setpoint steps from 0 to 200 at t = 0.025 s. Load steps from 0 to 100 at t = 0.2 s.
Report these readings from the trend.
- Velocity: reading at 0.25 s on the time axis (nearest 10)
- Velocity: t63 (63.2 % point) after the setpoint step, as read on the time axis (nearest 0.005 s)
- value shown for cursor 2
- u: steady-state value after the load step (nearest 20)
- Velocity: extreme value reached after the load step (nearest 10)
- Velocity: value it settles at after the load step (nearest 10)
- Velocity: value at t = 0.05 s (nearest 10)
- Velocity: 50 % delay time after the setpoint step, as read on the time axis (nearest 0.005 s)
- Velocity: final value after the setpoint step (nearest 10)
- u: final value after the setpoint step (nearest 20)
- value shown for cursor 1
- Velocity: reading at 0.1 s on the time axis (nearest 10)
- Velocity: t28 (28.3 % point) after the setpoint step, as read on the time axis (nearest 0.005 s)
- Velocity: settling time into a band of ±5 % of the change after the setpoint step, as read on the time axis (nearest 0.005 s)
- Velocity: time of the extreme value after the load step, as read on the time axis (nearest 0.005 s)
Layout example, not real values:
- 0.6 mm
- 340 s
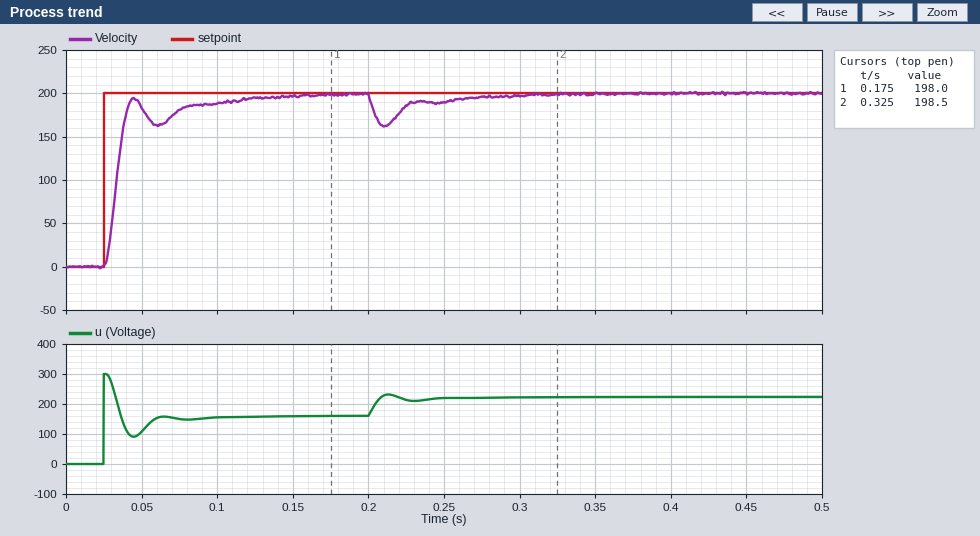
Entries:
- 190
- 0.035 s
- 198.5
- 220
- 160
- 200
- 180
- 0.035 s
- 200
- 160
- 198.0
- 190
- 0.030 s
- 0.105 s
- 0.210 s
